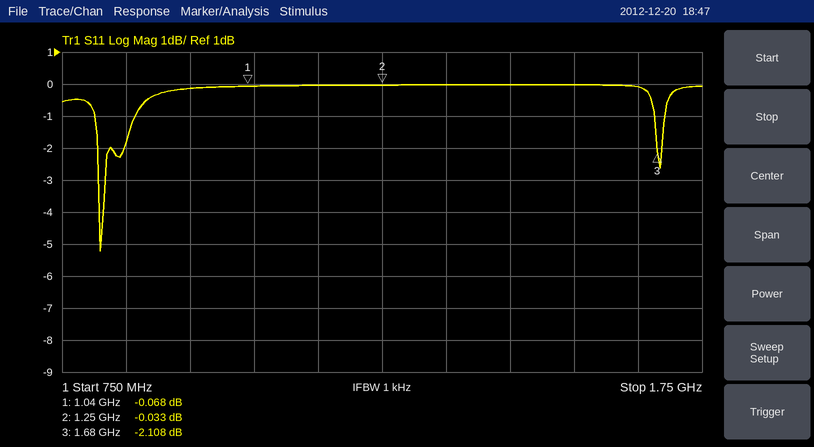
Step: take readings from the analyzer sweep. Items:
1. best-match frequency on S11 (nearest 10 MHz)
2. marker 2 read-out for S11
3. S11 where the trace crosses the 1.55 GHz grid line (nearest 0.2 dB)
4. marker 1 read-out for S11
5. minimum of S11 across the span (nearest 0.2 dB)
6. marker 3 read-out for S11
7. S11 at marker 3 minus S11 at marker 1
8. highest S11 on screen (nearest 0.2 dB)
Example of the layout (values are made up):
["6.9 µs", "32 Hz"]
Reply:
["810 MHz", "-0.033 dB", "0.0 dB", "-0.068 dB", "-5.2 dB", "-2.108 dB", "-2.040 dB", "0.0 dB"]
